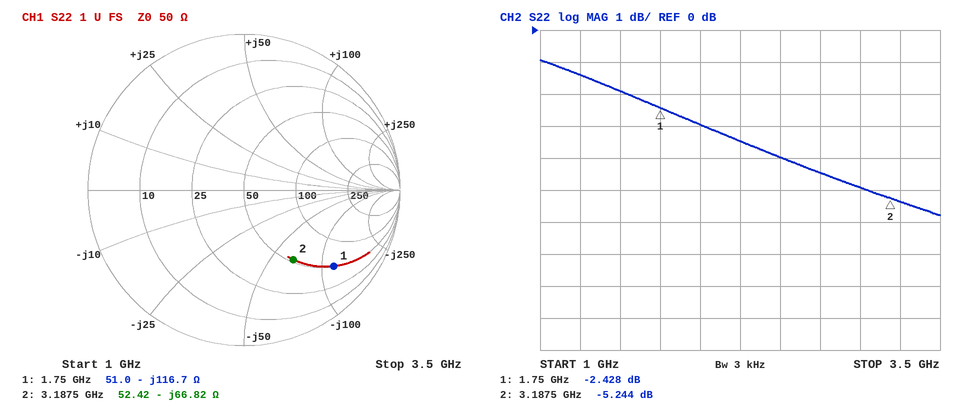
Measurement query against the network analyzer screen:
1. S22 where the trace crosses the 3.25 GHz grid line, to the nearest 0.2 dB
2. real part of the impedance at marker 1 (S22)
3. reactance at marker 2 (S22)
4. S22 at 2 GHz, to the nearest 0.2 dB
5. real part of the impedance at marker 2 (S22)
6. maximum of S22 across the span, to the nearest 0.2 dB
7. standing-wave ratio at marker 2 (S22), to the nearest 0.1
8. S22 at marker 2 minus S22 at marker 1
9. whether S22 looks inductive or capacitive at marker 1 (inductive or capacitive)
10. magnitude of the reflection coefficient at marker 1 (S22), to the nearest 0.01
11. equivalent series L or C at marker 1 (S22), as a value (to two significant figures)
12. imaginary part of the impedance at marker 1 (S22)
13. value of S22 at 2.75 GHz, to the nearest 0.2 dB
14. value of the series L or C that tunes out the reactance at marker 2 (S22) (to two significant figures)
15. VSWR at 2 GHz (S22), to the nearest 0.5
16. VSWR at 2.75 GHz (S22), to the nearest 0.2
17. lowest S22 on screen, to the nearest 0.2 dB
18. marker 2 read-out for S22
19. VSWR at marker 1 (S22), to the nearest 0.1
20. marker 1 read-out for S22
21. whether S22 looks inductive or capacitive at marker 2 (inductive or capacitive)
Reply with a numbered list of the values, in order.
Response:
1. -5.4 dB
2. 51.0 Ω
3. -66.82 Ω
4. -3.0 dB
5. 52.42 Ω
6. -1.0 dB
7. 3.4
8. -2.816 dB
9. capacitive
10. 0.76
11. 780 fF
12. -116.7 Ω
13. -4.4 dB
14. 3.3 nH
15. 6.0
16. 4.0
17. -5.8 dB
18. -5.244 dB
19. 7.2
20. -2.428 dB
21. capacitive
